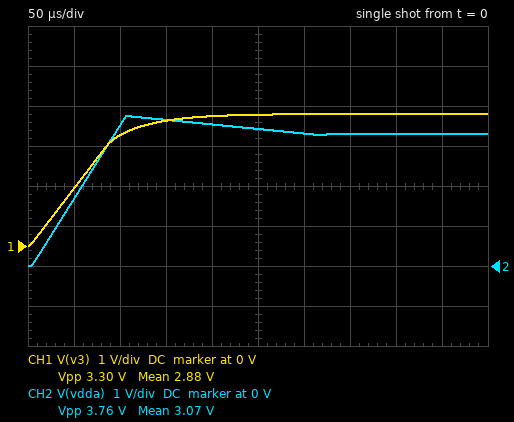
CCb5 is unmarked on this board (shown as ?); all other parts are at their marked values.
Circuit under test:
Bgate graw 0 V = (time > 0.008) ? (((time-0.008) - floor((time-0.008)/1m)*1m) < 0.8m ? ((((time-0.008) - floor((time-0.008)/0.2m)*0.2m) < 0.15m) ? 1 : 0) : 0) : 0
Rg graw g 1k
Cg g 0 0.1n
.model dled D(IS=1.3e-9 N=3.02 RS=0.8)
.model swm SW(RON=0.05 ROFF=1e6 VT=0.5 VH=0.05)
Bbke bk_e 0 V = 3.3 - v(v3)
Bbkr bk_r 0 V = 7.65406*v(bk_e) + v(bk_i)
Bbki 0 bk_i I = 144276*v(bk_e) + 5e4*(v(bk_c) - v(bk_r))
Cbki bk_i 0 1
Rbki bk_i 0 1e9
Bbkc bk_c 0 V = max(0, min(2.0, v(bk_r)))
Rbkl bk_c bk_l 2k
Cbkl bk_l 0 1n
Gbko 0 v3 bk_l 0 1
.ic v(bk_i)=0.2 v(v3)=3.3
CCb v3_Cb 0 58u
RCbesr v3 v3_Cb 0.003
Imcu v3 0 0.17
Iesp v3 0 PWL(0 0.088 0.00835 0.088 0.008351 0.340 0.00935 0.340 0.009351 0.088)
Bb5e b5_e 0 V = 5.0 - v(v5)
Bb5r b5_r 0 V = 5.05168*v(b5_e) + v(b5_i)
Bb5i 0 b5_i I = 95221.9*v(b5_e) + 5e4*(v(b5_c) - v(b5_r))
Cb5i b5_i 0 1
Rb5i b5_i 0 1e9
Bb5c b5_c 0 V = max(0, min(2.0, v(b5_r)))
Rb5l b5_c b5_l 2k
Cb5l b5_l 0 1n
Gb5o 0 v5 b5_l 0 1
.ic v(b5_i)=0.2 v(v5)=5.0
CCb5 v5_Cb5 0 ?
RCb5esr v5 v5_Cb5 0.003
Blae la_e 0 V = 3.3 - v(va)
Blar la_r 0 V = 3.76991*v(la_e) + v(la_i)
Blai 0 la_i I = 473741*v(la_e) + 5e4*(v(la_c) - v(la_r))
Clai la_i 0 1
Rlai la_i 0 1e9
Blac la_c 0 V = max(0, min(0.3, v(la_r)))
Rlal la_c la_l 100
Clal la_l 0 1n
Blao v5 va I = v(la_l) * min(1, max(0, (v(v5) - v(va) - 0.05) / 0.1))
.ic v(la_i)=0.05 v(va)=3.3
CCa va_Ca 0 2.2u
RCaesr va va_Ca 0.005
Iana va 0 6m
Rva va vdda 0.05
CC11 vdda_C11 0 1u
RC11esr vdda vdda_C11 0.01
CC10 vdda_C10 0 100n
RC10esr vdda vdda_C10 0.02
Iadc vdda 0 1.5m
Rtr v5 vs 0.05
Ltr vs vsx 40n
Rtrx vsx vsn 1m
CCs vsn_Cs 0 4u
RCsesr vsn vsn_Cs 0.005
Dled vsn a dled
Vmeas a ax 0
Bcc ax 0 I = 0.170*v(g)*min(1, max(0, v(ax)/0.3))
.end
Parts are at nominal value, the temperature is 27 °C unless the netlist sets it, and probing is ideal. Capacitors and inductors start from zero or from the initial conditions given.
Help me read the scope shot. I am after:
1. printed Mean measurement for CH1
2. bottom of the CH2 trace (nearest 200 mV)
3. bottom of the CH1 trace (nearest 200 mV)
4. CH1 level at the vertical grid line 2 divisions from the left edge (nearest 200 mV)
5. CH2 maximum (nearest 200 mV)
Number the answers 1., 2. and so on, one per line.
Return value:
1. 2.88 V
2. 0 V
3. 0 V
4. 2.8 V
5. 3.8 V
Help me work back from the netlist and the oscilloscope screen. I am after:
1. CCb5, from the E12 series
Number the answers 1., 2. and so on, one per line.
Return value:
1. 47 µF
